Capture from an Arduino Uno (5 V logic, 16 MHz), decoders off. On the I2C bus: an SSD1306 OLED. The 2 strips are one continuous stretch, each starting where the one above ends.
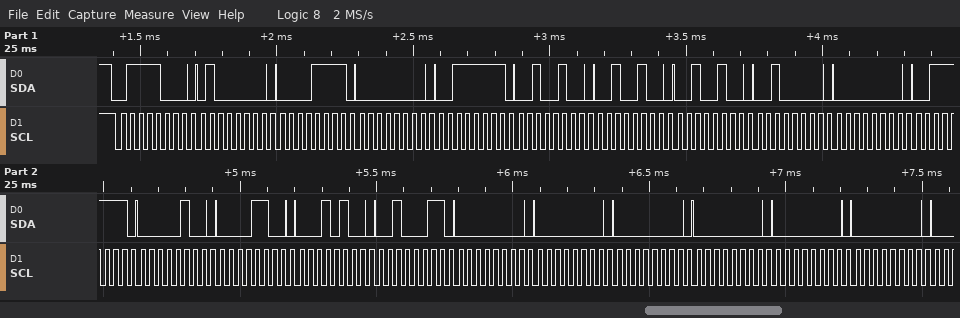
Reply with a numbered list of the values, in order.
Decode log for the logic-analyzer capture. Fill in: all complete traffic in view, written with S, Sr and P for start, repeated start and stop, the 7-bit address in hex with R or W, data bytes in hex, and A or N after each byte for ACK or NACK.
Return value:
1. S 3CW A 40 A 0F A 00 A 3F A 24 A 24 A 24 A 20 A 00 A 3F A 04 A 0C A 14 A 23 A 00 A 00 A 00 A 00 A 00 A 00 A
